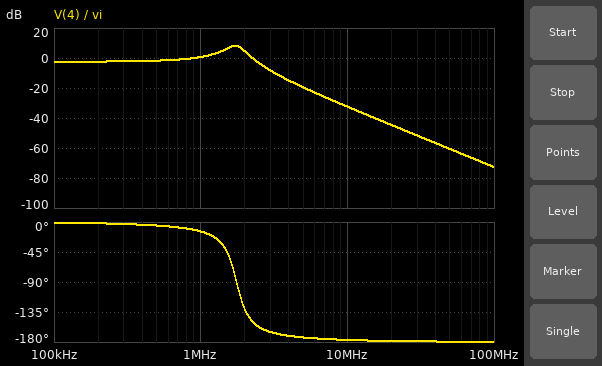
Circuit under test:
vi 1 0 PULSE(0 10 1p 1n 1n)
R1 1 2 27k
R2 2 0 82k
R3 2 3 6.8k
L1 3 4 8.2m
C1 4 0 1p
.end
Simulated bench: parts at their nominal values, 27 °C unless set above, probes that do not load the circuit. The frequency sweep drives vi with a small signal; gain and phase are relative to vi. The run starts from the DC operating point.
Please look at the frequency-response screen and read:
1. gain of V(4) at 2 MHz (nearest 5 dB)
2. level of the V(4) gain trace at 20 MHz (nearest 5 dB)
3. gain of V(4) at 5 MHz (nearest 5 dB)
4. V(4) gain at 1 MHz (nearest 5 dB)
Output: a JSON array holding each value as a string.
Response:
["5 dB", "-45 dB", "-20 dB", "0 dB"]
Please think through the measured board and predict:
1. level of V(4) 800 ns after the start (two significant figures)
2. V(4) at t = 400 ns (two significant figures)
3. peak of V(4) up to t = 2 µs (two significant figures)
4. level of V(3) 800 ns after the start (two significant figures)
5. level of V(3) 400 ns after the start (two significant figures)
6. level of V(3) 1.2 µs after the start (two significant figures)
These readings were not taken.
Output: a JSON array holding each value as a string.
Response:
["8.9 V", "9.4 V", "12 V", "7.1 V", "8.6 V", "7.4 V"]
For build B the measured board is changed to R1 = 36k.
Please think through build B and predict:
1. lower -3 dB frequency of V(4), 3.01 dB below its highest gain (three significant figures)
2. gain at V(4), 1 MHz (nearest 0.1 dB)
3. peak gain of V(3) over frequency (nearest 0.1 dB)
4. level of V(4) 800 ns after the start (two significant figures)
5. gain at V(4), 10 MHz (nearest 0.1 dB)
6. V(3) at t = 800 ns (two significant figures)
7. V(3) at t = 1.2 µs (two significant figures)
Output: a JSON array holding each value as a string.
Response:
["1.35 MHz", "-0.1 dB", "-3.2 dB", "7.9 V", "-33.1 dB", "6.6 V", "6.8 V"]
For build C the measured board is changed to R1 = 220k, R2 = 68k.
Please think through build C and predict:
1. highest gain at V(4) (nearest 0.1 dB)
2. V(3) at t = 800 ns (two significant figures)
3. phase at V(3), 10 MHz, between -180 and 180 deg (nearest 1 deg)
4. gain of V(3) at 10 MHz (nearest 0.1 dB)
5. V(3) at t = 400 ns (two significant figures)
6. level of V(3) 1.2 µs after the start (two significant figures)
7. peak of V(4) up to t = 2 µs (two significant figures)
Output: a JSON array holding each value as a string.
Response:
["-8.3 dB", "2.3 V", "7 deg", "-12.6 dB", "2.7 V", "2.4 V", "3.2 V"]
